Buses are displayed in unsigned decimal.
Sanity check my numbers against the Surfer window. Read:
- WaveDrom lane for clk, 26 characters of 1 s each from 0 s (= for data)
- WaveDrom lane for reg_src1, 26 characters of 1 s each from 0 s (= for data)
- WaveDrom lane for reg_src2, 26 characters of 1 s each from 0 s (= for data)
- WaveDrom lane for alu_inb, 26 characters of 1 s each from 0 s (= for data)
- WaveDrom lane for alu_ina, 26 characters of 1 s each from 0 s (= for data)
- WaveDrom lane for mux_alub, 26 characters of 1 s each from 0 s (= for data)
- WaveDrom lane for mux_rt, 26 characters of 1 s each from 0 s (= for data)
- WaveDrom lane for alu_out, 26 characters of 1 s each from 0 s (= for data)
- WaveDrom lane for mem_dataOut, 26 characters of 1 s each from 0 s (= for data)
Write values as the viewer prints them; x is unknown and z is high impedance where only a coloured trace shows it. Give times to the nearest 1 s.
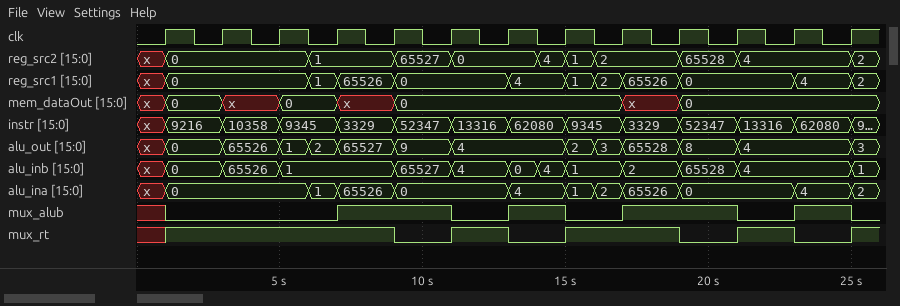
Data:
{name: 'clk', wave: '01010101010101010101010101'}
{name: 'reg_src1', wave: 'x=....==.=...=.===.=...=.=', data: '0 1 65526 0 4 1 2 65526 0 4 2'}
{name: 'reg_src2', wave: 'x=....=..=.=..===..=.=...=', data: '0 1 65527 0 4 1 2 65528 4 2'}
{name: 'alu_inb', wave: 'x=.=.=...=.=.===.=.=.=...=', data: '0 65526 1 65527 4 0 4 1 2 65528 4 1'}
{name: 'alu_ina', wave: 'x=....==.=...=.===.=...=.=', data: '0 1 65526 0 4 1 2 65526 0 4 2'}
{name: 'mux_alub', wave: 'x0.....1...0.1.0.1...0.1.0'}
{name: 'mux_rt', wave: 'x1.......0.1.0.1...0.1.0.1'}
{name: 'alu_out', wave: 'x=.=.===.=.=...===.=.=...=', data: '0 65526 1 2 65527 9 4 2 3 65528 8 4 3'}
{name: 'mem_dataOut', wave: 'x=.x.=.x.=.......x.=......', data: '0 0 0 0'}
